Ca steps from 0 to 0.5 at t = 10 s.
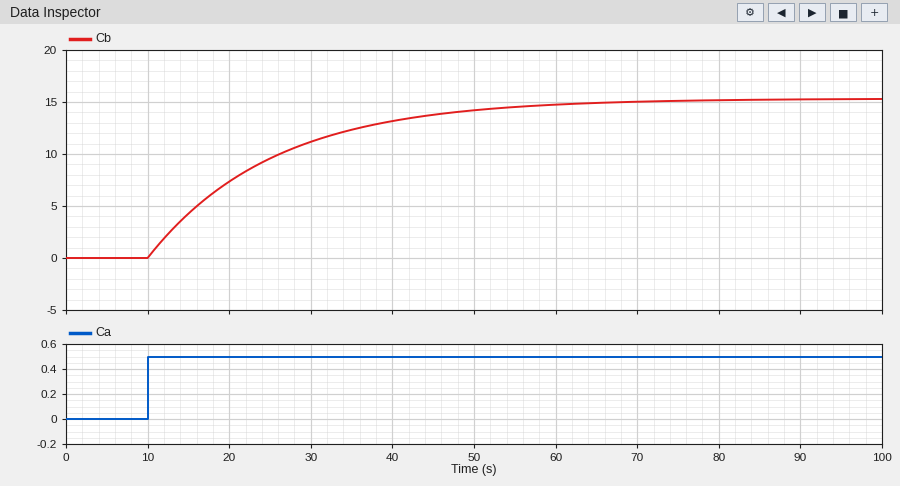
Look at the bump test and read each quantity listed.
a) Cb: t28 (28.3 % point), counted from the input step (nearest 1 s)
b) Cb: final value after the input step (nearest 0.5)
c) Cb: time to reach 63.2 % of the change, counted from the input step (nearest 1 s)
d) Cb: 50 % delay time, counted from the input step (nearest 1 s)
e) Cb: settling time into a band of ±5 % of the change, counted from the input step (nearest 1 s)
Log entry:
5 s
15.5
15 s
11 s
46 s
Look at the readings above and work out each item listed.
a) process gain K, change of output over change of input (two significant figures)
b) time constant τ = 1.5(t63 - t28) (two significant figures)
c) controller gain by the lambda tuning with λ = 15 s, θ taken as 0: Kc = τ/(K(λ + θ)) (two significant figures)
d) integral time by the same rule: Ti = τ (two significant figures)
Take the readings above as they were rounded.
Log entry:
31
15 s
0.032
15 s
